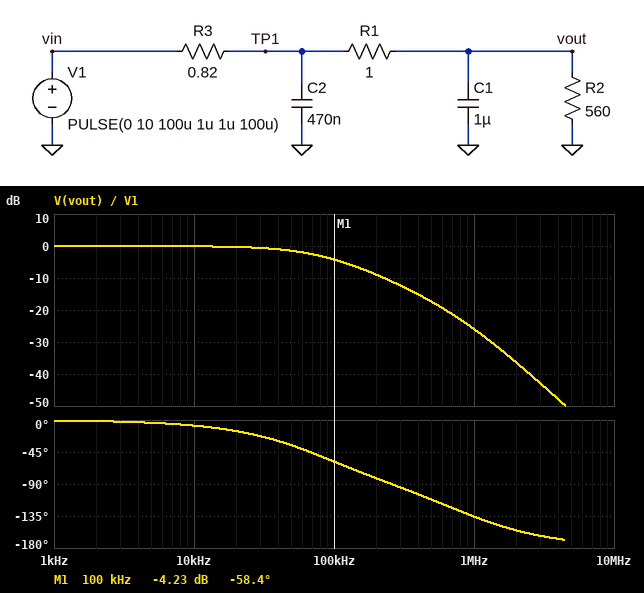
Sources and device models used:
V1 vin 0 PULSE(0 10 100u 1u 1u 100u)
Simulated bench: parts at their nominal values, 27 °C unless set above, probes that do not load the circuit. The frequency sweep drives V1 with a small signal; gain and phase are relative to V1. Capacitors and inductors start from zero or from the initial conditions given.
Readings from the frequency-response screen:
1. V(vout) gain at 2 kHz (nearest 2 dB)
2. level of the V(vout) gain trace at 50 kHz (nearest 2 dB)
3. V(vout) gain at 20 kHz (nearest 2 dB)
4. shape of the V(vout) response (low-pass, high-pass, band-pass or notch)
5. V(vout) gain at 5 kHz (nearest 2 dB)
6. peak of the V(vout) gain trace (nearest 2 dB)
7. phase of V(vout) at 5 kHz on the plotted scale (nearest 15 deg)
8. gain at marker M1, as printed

0 dB
-2 dB
0 dB
low-pass
0 dB
0 dB
0 deg
-4.23 dB
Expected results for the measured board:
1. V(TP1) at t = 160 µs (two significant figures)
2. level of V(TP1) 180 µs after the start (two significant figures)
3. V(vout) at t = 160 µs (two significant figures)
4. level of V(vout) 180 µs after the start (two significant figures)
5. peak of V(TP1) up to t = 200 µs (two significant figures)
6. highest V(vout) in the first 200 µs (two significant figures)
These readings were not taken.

10 V
10 V
10 V
10 V
10 V
10 V
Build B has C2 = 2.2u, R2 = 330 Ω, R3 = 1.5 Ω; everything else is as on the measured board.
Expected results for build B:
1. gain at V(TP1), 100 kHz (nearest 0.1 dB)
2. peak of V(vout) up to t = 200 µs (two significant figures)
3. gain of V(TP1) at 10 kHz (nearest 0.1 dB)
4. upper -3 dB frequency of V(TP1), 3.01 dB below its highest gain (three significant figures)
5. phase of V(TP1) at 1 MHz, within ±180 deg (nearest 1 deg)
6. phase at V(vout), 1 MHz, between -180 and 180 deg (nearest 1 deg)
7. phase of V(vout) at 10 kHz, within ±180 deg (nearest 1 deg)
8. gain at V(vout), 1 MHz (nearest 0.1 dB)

-9.8 dB
9.9 V
-0.5 dB
31.7 kHz
-83 deg
-164 deg
-20 deg
-42.6 dB
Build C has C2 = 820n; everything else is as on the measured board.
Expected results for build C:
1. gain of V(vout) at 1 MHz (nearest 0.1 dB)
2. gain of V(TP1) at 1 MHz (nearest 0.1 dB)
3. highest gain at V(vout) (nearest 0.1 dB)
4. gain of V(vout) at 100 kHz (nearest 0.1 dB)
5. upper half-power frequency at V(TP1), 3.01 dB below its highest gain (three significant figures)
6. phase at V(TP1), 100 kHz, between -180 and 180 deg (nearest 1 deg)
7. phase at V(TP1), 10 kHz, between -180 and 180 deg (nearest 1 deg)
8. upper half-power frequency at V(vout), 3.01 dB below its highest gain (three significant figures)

-29.5 dB
-13.5 dB
0 dB
-4.8 dB
92.0 kHz
-33 deg
-5 deg
71.7 kHz
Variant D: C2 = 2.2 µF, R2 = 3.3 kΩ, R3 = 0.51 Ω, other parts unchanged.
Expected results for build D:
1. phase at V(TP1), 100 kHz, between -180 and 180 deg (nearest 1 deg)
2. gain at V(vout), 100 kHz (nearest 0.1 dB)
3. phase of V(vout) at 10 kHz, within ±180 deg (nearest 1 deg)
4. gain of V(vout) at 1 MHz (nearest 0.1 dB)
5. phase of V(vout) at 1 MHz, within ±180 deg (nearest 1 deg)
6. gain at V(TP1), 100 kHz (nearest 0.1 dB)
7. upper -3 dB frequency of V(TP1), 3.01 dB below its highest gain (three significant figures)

-39 deg
-4.8 dB
-9 deg
-33.3 dB
-159 deg
-3.4 dB
90.6 kHz
